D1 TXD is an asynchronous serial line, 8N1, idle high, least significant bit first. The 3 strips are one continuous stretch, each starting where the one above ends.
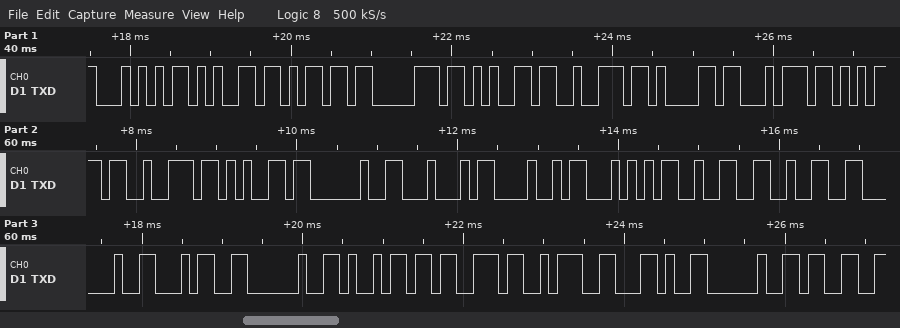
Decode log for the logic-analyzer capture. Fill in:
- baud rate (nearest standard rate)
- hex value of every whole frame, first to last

9600 baud
0x54 0x65 0x6D 0x70 0x65 0x72 0x61 0x74 0x75 0x72 0x65 0x20 0x44 0x48 0x54 0x32 0x32 0x20 0x34 0x20 0x69 0x73 0x3A 0x2C 0x20 0x33
